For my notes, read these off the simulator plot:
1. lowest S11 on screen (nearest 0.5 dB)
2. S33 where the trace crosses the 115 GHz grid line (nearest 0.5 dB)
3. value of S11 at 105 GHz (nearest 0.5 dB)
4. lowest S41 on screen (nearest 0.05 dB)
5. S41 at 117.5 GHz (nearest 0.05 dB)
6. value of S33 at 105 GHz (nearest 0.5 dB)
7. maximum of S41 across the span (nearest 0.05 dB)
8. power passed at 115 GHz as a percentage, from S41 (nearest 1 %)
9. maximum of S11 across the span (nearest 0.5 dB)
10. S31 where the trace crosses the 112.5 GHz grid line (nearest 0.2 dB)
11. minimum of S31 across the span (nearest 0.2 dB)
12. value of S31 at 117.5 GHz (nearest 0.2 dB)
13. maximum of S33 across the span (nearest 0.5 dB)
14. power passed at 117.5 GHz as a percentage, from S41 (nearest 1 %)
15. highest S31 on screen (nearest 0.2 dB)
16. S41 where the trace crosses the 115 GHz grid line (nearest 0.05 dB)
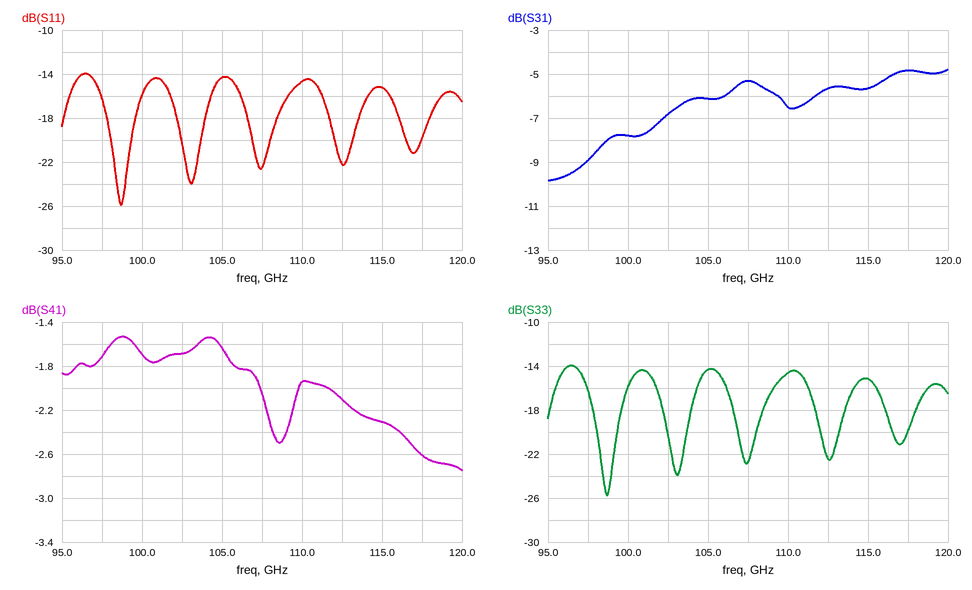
-26.0 dB
-15.0 dB
-14.5 dB
-2.75 dB
-2.60 dB
-14.5 dB
-1.55 dB
59 %
-14.0 dB
-5.6 dB
-9.8 dB
-4.8 dB
-14.0 dB
55 %
-4.8 dB
-2.30 dB
